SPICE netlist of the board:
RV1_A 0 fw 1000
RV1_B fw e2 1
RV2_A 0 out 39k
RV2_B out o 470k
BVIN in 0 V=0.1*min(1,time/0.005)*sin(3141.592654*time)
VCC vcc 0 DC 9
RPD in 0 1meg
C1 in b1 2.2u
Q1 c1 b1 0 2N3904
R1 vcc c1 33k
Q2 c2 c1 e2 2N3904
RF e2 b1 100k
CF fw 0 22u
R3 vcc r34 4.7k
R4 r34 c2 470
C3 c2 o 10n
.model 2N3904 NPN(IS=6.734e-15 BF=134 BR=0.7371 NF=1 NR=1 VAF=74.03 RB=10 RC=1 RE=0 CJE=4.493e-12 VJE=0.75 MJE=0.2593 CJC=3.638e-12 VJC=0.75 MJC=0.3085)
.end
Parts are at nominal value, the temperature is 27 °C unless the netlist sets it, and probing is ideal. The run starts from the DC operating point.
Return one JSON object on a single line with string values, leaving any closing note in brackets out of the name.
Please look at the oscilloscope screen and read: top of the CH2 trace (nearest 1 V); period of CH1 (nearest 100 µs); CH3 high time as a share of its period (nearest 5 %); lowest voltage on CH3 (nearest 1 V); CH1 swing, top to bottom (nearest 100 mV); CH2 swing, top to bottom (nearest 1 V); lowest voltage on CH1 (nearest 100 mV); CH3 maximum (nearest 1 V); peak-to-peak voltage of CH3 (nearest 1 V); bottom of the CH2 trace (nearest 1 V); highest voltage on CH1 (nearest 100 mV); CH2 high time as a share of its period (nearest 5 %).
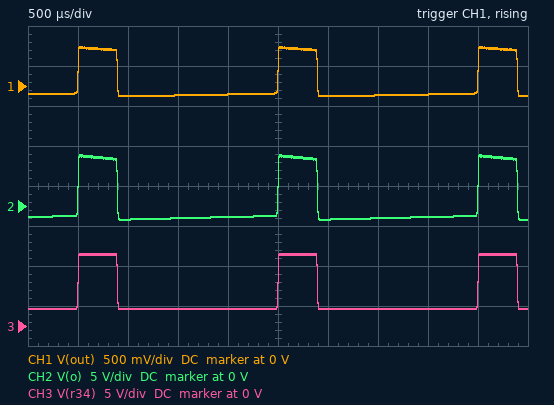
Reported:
{"top of the CH2 trace": "6 V", "period of CH1": "2.0 ms", "CH3 high time as a share of its period": "20 %", "lowest voltage on CH3": "2 V", "CH1 swing, top to bottom": "600 mV", "CH2 swing, top to bottom": "8 V", "lowest voltage on CH1": "-100 mV", "CH3 maximum": "9 V", "peak-to-peak voltage of CH3": "7 V", "bottom of the CH2 trace": "-2 V", "highest voltage on CH1": "500 mV", "CH2 high time as a share of its period": "20 %"}
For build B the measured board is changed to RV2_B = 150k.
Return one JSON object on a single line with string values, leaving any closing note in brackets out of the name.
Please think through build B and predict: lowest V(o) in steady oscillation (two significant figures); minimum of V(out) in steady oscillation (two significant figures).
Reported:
{"lowest V(o) in steady oscillation": "-2.1 V", "minimum of V(out) in steady oscillation": "-430 mV"}
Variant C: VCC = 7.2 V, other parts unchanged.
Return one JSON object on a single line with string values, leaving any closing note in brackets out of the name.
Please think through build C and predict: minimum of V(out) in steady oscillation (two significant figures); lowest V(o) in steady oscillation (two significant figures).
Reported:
{"minimum of V(out) in steady oscillation": "-100 mV", "lowest V(o) in steady oscillation": "-1.3 V"}
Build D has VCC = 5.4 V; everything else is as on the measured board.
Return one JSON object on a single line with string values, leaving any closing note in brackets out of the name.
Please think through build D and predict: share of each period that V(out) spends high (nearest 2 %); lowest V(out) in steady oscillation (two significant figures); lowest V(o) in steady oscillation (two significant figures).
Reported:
{"share of each period that V(out) spends high": "18 %", "lowest V(out) in steady oscillation": "-72 mV", "lowest V(o) in steady oscillation": "-940 mV"}
